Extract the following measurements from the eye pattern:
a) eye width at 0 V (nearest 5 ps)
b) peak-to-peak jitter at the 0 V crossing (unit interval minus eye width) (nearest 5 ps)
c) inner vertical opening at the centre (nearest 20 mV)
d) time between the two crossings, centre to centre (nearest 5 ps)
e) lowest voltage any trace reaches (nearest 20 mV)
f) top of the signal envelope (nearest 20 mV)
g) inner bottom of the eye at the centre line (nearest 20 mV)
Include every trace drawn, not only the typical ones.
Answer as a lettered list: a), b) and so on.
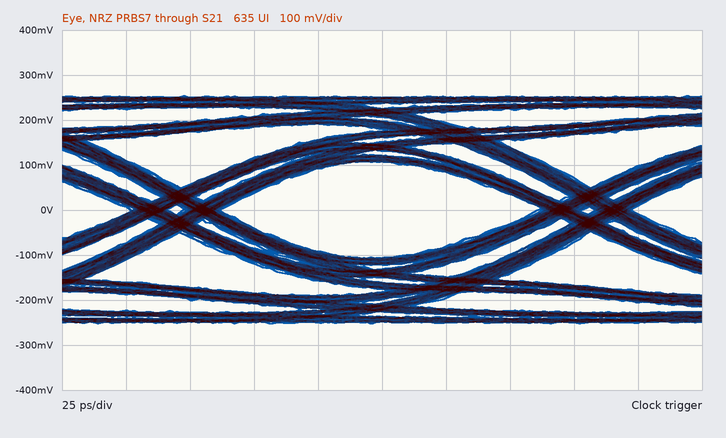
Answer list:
a) 125 ps
b) 35 ps
c) 220 mV
d) 160 ps
e) -260 mV
f) 260 mV
g) -100 mV
